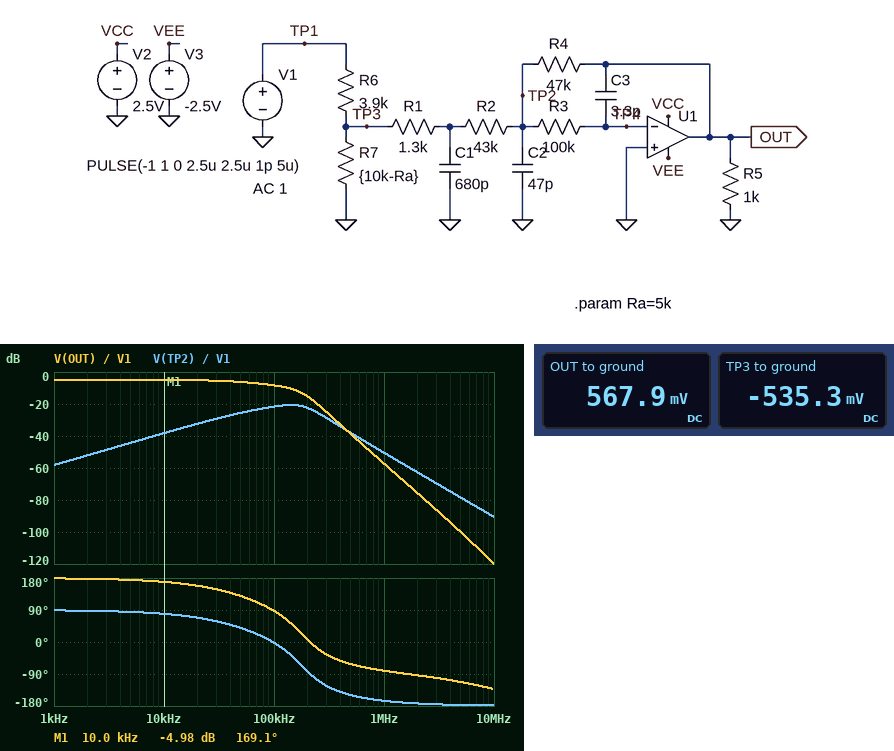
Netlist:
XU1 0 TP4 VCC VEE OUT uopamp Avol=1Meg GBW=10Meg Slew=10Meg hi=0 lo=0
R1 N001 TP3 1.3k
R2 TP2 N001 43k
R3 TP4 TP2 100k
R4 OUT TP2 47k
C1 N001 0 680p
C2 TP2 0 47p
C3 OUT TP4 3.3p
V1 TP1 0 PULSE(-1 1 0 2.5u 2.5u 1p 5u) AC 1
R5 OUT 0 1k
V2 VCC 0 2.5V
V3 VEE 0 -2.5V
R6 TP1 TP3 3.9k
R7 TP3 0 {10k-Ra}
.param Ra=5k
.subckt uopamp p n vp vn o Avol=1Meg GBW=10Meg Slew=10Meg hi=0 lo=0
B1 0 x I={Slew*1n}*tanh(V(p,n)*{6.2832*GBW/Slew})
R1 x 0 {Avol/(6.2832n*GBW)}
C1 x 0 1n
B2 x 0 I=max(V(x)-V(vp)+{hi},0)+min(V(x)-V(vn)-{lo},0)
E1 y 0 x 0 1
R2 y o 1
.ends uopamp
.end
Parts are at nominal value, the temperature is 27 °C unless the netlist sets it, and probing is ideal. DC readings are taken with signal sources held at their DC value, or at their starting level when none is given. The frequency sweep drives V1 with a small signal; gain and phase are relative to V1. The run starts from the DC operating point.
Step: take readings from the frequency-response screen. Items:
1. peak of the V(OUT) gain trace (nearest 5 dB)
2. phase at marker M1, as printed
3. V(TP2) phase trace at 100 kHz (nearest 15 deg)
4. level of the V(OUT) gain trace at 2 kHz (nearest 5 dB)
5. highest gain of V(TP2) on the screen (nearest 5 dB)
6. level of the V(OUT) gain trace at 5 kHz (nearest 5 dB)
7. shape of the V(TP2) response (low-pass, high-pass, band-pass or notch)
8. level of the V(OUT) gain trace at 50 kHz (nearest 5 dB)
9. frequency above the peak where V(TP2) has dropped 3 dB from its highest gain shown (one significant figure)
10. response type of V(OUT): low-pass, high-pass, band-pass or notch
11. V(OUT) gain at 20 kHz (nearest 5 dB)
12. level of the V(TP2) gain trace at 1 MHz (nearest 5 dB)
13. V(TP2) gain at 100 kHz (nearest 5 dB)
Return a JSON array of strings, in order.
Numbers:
["-5 dB", "169.1 deg", "0 deg", "-5 dB", "-20 dB", "-5 dB", "band-pass", "-5 dB", "200 kHz", "low-pass", "-5 dB", "-50 dB", "-20 dB"]
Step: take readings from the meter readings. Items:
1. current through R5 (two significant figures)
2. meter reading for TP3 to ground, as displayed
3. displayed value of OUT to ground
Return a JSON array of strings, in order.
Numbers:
["570 µA", "-535.3 mV", "567.9 mV"]
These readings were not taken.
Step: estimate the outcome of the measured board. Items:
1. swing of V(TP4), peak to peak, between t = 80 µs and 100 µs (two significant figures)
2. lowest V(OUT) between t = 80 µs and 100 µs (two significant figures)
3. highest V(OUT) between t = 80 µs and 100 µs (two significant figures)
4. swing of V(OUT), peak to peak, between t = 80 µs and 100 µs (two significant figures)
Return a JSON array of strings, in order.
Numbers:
["5.7 mV", "-140 mV", "140 mV", "280 mV"]
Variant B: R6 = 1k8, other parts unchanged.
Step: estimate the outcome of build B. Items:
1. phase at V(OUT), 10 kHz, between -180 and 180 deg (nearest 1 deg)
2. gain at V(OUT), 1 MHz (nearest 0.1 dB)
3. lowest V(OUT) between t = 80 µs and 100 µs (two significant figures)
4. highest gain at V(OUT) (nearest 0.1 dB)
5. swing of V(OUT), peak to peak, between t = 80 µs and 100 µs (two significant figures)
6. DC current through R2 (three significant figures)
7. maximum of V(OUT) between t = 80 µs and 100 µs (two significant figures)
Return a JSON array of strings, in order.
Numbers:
["171 deg", "-52.4 dB", "-240 mV", "-2.4 dB", "480 mV", "16.1 µA", "240 mV"]
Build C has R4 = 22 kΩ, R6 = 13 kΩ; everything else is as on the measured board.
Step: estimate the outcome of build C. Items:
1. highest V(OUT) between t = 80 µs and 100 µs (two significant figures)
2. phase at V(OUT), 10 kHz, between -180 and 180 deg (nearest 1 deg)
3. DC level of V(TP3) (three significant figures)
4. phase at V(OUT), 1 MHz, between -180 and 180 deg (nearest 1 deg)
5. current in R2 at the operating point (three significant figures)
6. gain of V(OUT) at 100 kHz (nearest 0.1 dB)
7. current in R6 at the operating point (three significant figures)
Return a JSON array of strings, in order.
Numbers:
["31 mV", "167 deg", "-257 mV", "-77 deg", "5.80 µA", "-23.8 dB", "57.2 µA"]
